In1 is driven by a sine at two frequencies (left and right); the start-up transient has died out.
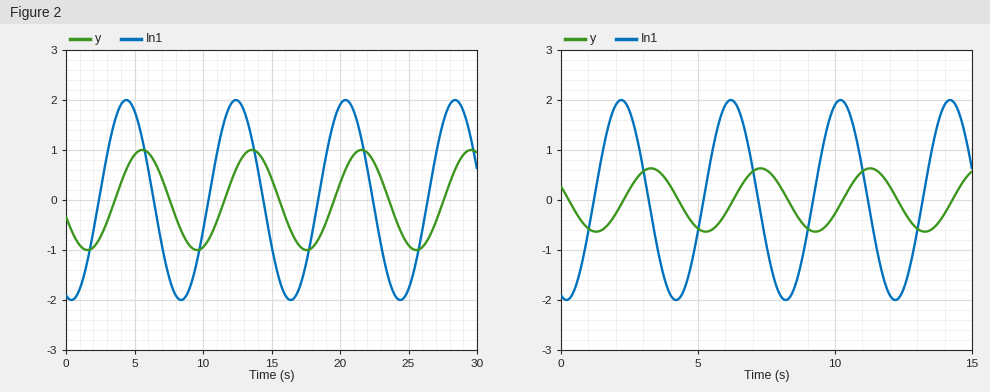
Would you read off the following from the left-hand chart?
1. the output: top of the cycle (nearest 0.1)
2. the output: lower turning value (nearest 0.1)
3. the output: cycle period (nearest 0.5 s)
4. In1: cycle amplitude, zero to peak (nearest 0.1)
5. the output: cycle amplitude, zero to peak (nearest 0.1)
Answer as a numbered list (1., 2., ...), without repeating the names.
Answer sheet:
1. 1.0
2. -1.0
3. 8.0 s
4. 2.0
5. 1.0
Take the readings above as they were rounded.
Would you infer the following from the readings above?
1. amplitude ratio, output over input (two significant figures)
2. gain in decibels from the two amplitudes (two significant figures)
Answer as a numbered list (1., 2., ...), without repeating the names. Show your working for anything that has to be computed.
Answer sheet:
1. 1 / 2 = 0.50
2. 20 log10(1 / 2) = -6.0 dB
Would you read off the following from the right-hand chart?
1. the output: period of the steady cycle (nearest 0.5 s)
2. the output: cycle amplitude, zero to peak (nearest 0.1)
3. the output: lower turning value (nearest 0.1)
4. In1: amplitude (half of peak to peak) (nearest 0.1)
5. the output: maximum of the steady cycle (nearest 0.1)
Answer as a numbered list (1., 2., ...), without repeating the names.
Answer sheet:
1. 4.0 s
2. 0.6
3. -0.6
4. 2.0
5. 0.6
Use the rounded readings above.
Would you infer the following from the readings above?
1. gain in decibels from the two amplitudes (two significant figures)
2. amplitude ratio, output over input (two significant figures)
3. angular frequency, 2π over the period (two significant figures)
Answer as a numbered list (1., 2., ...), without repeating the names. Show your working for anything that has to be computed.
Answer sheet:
1. 20 log10(0.6 / 2) = -10 dB
2. 0.6 / 2 = 0.30
3. 2π / 4 = 1.6 rad/s
